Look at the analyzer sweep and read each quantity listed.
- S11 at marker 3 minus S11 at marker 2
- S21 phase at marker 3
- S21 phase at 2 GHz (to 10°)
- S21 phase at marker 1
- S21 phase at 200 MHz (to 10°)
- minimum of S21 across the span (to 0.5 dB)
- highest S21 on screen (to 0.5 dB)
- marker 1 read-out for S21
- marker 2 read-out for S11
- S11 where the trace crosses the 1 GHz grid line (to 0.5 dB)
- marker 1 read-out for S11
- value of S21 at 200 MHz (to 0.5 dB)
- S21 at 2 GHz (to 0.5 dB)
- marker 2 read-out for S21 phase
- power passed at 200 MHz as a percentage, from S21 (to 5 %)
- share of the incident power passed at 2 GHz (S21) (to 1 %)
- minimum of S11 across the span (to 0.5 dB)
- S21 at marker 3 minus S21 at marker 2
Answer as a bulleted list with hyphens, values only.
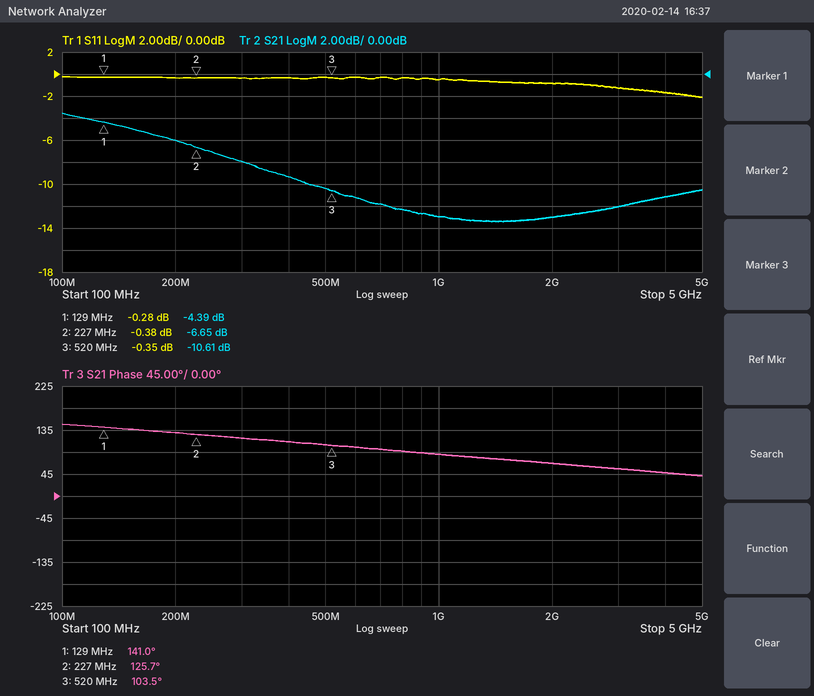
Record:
- 0.03 dB
- 103.5°
- 70°
- 141.0°
- 130°
- -13.5 dB
- -3.5 dB
- -4.39 dB
- -0.38 dB
- -0.5 dB
- -0.28 dB
- -6.0 dB
- -13.0 dB
- 125.7°
- 25 %
- 5 %
- -2.0 dB
- -3.96 dB
